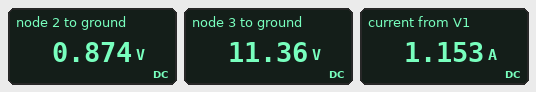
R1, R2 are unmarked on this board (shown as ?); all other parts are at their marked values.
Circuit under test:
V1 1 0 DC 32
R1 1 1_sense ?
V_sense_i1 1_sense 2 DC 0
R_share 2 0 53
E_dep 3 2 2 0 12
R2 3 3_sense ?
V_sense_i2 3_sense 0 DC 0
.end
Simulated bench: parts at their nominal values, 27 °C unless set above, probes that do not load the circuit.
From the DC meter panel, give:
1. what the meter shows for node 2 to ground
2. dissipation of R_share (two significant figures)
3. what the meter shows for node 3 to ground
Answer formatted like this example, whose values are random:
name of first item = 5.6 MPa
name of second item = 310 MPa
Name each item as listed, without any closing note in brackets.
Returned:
what the meter shows for node 2 to ground = 0.874 V
dissipation of R_share = 14 mW
what the meter shows for node 3 to ground = 11.36 V
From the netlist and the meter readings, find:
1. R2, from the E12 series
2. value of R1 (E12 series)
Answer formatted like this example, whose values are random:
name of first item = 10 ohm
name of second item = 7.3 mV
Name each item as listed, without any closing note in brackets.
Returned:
R2, from the E12 series = 10 Ω
value of R1 = 27 Ω
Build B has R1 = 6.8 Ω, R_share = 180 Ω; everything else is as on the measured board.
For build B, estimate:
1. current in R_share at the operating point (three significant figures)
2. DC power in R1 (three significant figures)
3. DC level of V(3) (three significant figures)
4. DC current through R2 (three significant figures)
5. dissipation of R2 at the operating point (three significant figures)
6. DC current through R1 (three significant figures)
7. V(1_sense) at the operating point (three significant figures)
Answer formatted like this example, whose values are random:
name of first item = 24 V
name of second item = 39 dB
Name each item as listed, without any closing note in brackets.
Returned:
current in R_share at the operating point = 18.0 mA
DC power in R1 = 122 W
DC level of V(3) = 42.1 V
DC current through R2 = 4.21 A
dissipation of R2 at the operating point = 177 W
DC current through R1 = 4.23 A
V(1_sense) at the operating point = 3.24 V
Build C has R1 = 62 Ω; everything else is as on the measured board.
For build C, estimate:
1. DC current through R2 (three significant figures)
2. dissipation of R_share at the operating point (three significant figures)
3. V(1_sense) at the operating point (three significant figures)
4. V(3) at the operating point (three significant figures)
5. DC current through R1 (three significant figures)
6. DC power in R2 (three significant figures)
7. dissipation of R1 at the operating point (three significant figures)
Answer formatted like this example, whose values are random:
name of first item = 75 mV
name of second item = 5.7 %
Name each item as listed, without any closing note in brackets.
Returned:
DC current through R2 = 503 mA
dissipation of R_share at the operating point = 2.82 mW
V(1_sense) at the operating point = 387 mV
V(3) at the operating point = 5.03 V
DC current through R1 = 510 mA
DC power in R2 = 2.53 W
dissipation of R1 at the operating point = 16.1 W
